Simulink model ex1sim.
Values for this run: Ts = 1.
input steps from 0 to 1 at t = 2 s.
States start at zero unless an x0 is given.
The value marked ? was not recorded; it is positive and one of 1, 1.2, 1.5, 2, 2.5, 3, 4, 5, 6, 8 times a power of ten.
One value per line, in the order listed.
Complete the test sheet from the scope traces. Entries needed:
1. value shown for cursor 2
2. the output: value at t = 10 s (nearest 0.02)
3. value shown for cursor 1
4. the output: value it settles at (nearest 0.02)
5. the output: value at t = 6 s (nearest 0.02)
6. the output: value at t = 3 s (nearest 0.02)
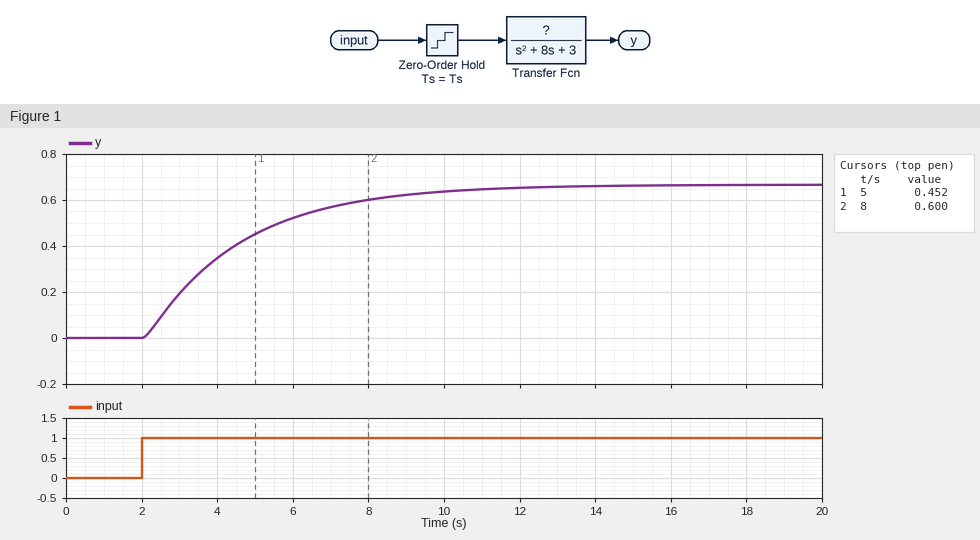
0.600
0.64
0.452
0.66
0.52
0.20
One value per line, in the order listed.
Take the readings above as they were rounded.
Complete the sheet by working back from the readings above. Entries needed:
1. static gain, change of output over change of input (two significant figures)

0.66
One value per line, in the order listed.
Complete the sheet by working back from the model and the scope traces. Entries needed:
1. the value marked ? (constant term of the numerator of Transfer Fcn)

2
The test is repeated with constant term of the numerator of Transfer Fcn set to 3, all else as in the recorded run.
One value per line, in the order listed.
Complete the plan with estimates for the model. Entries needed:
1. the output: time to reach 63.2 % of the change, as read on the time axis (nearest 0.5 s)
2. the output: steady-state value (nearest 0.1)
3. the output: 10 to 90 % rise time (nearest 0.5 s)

4.5 s
1.0
5.5 s
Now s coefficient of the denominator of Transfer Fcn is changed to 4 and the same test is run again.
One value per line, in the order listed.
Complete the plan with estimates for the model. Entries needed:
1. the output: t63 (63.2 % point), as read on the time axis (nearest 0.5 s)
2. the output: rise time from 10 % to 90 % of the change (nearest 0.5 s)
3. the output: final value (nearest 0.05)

3.5 s
2.5 s
0.65
